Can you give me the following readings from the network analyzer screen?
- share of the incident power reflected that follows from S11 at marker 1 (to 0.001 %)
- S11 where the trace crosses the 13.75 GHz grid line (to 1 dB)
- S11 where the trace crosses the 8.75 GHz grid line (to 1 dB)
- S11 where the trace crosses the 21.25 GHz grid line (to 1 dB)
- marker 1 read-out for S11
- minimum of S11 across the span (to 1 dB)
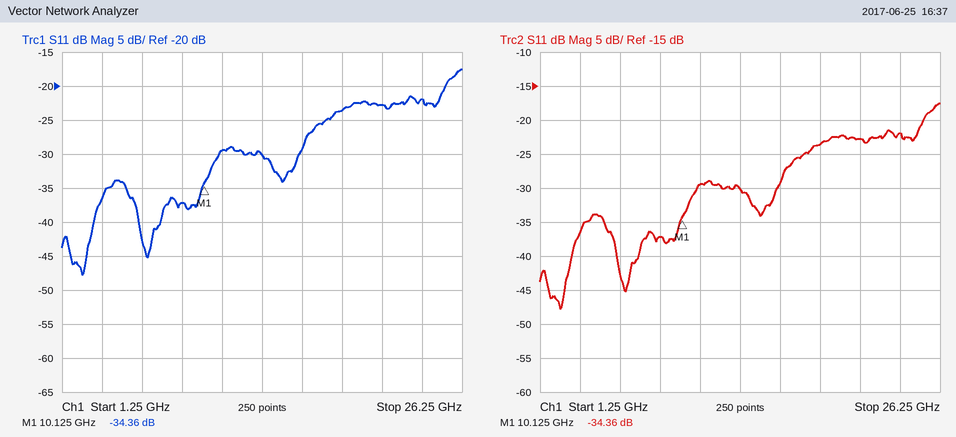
0.037 %
-30 dB
-37 dB
-23 dB
-34.36 dB
-48 dB
